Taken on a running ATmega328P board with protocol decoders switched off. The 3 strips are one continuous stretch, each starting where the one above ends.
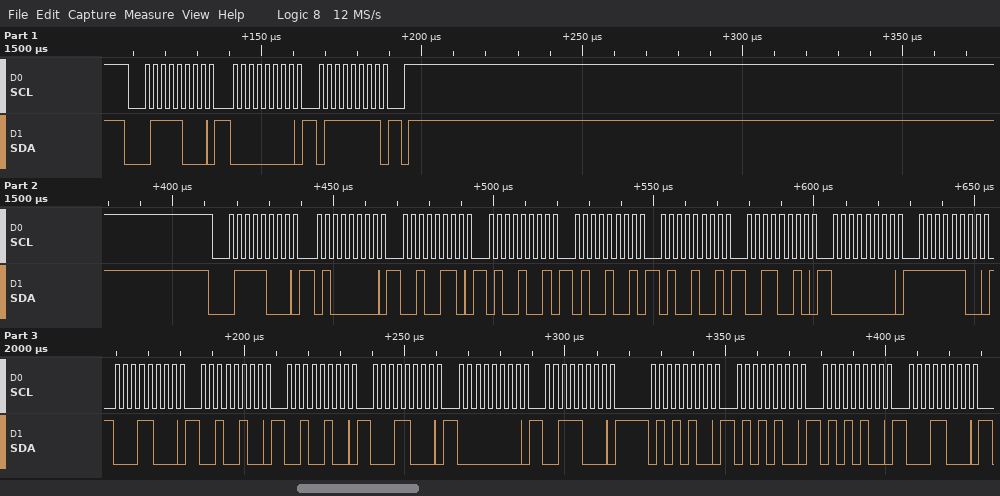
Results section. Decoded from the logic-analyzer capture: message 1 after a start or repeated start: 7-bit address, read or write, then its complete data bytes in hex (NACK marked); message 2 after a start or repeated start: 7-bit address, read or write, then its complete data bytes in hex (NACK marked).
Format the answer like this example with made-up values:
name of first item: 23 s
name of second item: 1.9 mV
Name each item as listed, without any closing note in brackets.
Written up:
message 1 after a start or repeated start: 7-bit address, read or write, then its complete data bytes in hex: 0x3C write: 00 7F
message 2 after a start or repeated start: 7-bit address, read or write, then its complete data bytes in hex: 0x3C write: 40 26 49 49 49 32 00 FC 18 24 24 18 00 38 54 54 54 18
